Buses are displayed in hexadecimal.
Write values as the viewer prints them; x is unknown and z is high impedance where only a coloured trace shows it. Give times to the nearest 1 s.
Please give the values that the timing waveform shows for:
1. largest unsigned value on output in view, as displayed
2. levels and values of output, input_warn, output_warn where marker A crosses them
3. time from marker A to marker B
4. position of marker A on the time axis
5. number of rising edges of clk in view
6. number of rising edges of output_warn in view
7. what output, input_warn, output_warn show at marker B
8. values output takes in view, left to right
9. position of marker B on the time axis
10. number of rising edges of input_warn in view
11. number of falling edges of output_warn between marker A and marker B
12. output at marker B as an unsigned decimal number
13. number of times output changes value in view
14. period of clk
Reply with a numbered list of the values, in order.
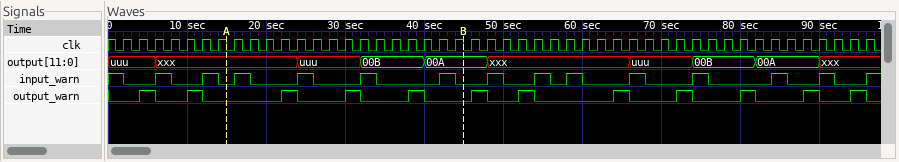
1. 00B
2. output=xxx, input_warn=0, output_warn=0
3. 30 s
4. 15 s
5. 48
6. 12
7. output=00A, input_warn=0, output_warn=0
8. uuu, xxx, uuu, 00B, 00A, xxx, uuu, 00B, 00A, xxx
9. 45 s
10. 14
11. 3
12. 10
13. 9
14. 2 s
